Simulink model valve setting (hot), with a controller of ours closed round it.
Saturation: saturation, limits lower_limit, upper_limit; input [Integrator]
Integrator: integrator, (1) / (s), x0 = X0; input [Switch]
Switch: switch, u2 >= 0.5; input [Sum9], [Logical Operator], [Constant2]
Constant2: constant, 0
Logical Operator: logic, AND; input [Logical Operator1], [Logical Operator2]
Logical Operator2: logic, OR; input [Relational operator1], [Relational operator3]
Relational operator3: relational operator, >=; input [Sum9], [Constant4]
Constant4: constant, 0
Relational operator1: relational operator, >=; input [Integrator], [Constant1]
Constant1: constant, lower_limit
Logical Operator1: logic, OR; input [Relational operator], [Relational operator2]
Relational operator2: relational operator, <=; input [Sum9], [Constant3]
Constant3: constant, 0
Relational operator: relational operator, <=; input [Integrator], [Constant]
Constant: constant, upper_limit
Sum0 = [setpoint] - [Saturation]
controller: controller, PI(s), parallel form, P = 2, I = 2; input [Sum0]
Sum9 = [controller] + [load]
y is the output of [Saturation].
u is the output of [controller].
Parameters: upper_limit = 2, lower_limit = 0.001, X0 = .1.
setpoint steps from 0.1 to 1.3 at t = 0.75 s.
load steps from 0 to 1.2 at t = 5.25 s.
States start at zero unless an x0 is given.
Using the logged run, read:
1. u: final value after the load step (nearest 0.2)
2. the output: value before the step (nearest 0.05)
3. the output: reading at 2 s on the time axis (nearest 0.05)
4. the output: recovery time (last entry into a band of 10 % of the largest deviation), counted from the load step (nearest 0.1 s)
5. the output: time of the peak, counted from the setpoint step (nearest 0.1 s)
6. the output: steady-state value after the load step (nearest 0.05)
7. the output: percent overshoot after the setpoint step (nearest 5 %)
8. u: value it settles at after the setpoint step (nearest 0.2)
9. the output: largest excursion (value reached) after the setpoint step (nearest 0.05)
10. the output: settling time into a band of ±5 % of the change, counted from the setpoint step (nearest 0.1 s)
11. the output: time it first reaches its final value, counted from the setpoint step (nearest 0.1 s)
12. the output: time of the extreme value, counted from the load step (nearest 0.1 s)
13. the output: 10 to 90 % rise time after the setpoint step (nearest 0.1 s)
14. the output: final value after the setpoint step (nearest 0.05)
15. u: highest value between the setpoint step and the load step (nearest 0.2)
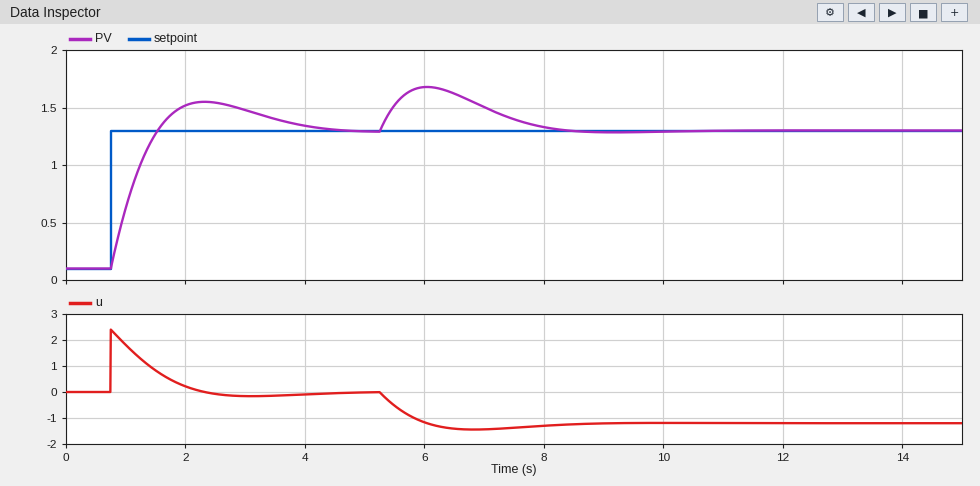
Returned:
-1.2
0.10
1.50
2.7 s
1.6 s
1.30
20 %
0.0
1.55
3.1 s
0.8 s
0.8 s
0.6 s
1.30
2.4
